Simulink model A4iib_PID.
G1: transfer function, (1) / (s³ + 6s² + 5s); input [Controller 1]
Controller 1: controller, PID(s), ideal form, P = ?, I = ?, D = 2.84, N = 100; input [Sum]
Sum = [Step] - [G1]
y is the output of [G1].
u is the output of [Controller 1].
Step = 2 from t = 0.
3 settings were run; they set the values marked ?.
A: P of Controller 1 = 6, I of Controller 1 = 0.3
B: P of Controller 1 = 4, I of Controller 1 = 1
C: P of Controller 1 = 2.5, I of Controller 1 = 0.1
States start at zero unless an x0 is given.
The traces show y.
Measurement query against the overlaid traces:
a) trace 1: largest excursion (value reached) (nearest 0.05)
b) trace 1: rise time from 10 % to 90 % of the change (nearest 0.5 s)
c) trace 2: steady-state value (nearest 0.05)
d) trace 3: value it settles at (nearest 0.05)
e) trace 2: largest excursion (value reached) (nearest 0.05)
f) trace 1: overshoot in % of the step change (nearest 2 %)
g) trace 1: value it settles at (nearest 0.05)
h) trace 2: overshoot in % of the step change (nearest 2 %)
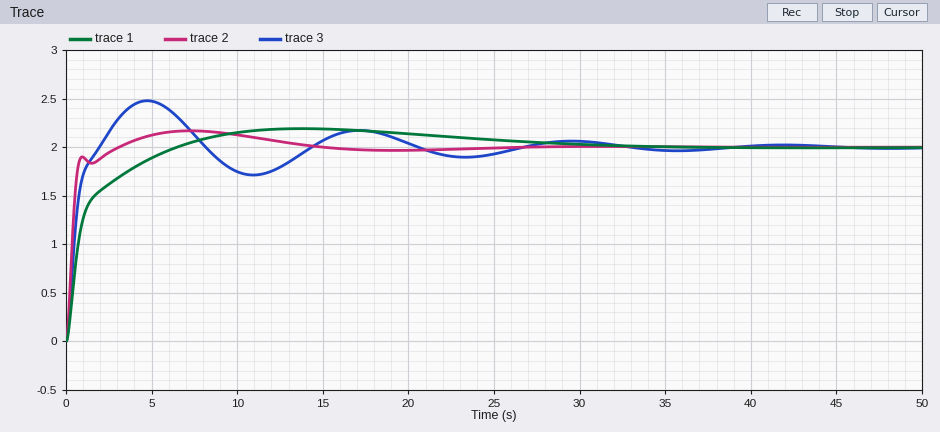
2.20
4.0 s
2.00
2.00
2.15
10 %
2.00
8 %
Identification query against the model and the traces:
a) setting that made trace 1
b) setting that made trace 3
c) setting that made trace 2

C
B
A
